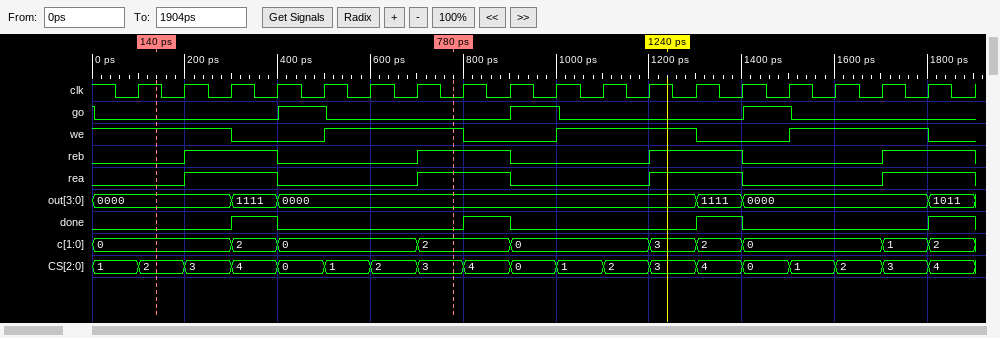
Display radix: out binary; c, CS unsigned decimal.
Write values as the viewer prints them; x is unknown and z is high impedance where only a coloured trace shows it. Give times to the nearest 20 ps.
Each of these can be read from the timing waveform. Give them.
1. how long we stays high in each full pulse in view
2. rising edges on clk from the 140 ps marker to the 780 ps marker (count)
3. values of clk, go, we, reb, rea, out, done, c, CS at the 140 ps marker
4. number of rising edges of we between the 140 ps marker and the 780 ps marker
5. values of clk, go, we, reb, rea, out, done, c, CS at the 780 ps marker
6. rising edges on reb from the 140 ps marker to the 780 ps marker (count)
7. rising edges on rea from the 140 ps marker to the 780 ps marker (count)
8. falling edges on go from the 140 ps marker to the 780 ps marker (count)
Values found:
300 ps, 300 ps, 300 ps
6
clk=1, go=0, we=1, reb=0, rea=0, out=0000, done=0, c=0, CS=2
1
clk=0, go=0, we=1, reb=1, rea=1, out=0000, done=0, c=2, CS=3
2
2
1
